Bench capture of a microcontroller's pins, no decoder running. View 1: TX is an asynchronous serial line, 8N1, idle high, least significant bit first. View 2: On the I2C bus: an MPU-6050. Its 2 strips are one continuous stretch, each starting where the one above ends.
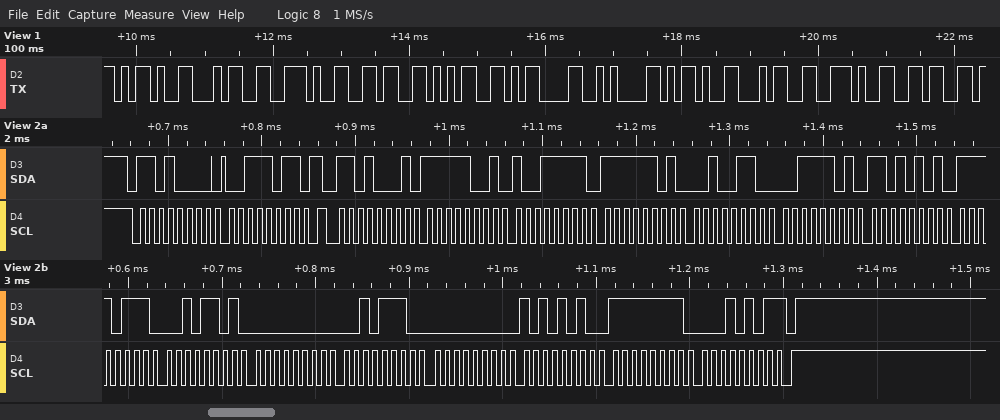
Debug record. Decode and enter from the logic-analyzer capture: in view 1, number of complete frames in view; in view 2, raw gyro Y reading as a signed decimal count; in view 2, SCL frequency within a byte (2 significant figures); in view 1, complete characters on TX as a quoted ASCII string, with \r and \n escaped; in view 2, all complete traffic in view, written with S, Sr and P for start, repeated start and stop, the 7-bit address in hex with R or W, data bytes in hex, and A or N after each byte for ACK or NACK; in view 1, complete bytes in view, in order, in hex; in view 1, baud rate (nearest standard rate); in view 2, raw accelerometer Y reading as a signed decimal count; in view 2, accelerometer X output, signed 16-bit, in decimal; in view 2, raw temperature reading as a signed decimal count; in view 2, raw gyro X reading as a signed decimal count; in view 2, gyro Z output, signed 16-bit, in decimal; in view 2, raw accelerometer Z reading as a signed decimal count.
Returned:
11
170
100 kHz
"-4.65\r\n-4.6"
S 68W A 3B A Sr 68R A F9 A 9F A FD A 26 A 3D A D5 A F7 A 2D A 00 A 2E A 00 A AA A FF A 15 N P
2D 34 2E 36 35 0D 0A 2D 34 2E 36
9600 baud
-730
-1633
-2259
46
-235
15829
